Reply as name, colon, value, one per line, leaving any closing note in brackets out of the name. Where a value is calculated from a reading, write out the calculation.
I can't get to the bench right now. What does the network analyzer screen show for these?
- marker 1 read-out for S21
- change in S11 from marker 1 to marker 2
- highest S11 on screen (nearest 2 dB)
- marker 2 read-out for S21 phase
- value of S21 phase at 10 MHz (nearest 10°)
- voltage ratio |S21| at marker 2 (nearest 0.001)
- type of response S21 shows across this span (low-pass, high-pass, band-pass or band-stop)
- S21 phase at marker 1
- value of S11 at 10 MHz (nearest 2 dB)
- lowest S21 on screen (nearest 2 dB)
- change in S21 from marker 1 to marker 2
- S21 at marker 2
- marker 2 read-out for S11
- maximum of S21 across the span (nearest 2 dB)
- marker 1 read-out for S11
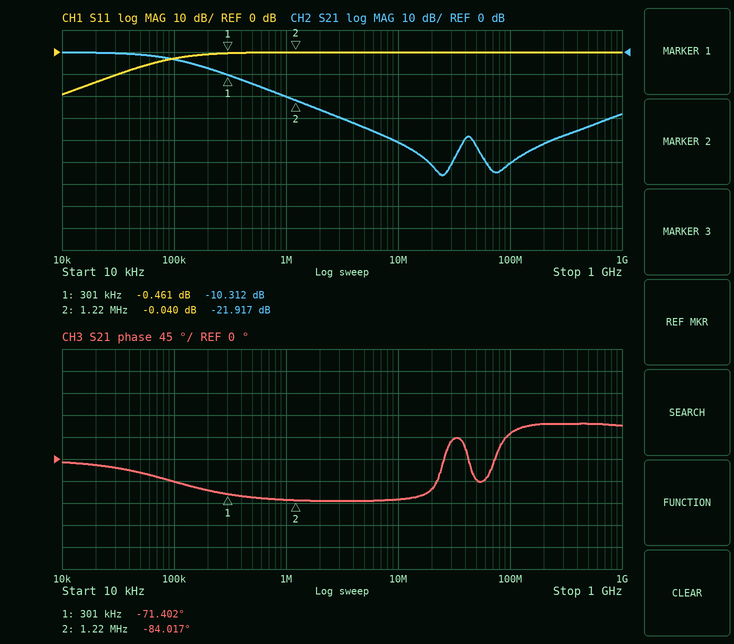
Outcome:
marker 1 read-out for S21: -10.312 dB
change in S11 from marker 1 to marker 2: -0.04 − (-0.461) = 0.421 dB
highest S11 on screen: 0 dB
marker 2 read-out for S21 phase: -84.017°
value of S21 phase at 10 MHz: -80°
voltage ratio |S21| at marker 2: 10^(-21.917/20) ≈ 0.080
type of response S21 shows across this span: low-pass
S21 phase at marker 1: -71.402°
value of S11 at 10 MHz: 0 dB
lowest S21 on screen: -56 dB
change in S21 from marker 1 to marker 2: -21.917 − (-10.312) = -11.605 dB
S21 at marker 2: -21.917 dB
marker 2 read-out for S11: -0.040 dB
maximum of S21 across the span: 0 dB
marker 1 read-out for S11: -0.461 dB
